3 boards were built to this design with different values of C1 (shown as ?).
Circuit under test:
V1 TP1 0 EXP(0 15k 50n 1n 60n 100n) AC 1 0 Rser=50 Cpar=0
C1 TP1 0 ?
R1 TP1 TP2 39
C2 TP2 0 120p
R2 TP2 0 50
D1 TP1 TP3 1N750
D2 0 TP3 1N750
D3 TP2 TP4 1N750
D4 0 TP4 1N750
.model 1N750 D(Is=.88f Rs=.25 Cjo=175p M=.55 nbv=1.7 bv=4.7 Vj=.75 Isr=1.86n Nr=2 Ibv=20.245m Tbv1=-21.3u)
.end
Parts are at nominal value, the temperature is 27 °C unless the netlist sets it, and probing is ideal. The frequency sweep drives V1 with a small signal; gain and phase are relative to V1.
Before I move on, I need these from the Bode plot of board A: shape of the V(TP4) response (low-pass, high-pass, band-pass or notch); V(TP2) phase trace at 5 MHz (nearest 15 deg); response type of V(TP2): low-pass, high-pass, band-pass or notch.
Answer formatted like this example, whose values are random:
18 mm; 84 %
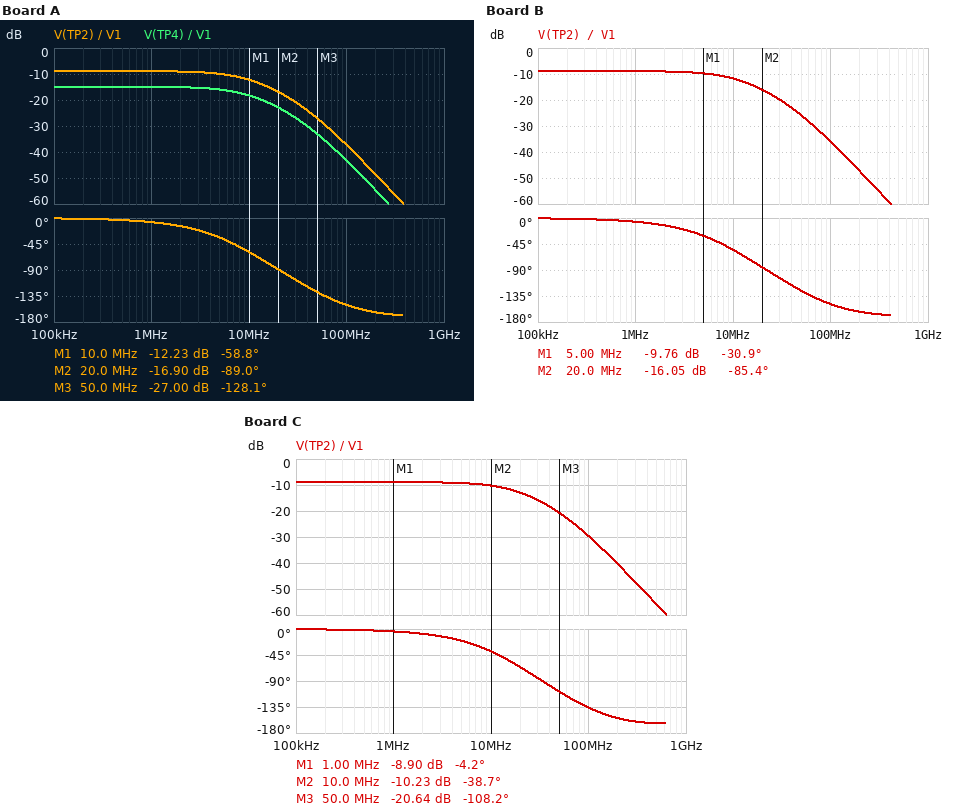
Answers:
low-pass; -30 deg; low-pass
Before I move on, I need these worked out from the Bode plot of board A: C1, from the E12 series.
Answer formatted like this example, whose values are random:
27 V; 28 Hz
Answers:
330 pF
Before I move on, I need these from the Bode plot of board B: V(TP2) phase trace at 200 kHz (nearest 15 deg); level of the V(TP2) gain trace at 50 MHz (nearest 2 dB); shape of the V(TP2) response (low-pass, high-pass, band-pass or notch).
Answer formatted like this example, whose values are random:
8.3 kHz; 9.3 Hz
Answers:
0 deg; -26 dB; low-pass
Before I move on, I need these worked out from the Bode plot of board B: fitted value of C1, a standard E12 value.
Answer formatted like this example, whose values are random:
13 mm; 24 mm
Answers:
270 pF
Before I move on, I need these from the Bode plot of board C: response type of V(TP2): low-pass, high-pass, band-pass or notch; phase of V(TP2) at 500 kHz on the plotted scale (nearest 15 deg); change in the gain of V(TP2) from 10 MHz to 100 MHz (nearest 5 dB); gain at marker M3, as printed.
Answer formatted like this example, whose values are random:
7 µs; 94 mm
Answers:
low-pass; 0 deg; -20 dB; -20.64 dB
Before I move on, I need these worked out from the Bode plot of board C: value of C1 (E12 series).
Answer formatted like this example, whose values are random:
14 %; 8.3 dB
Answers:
68 pF
